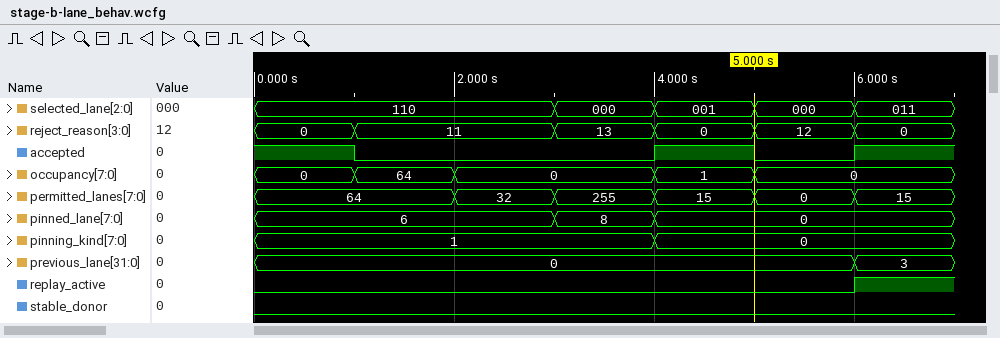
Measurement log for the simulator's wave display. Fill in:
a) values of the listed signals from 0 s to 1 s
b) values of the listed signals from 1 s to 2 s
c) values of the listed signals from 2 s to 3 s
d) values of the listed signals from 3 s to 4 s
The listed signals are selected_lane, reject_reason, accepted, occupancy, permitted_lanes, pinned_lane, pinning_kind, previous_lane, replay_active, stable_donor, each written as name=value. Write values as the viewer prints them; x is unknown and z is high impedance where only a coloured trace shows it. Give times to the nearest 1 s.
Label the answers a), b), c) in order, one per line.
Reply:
a) selected_lane=110, reject_reason=0, accepted=1, occupancy=0, permitted_lanes=64, pinned_lane=6, pinning_kind=1, previous_lane=0, replay_active=0, stable_donor=0
b) selected_lane=110, reject_reason=11, accepted=0, occupancy=64, permitted_lanes=64, pinned_lane=6, pinning_kind=1, previous_lane=0, replay_active=0, stable_donor=0
c) selected_lane=110, reject_reason=11, accepted=0, occupancy=0, permitted_lanes=32, pinned_lane=6, pinning_kind=1, previous_lane=0, replay_active=0, stable_donor=0
d) selected_lane=000, reject_reason=13, accepted=0, occupancy=0, permitted_lanes=255, pinned_lane=8, pinning_kind=1, previous_lane=0, replay_active=0, stable_donor=0
